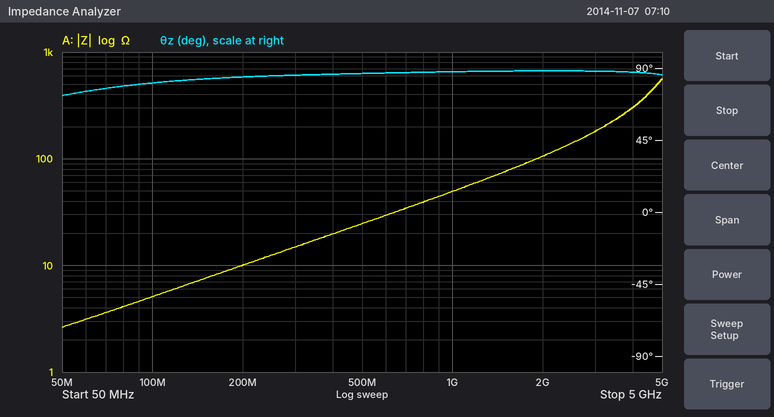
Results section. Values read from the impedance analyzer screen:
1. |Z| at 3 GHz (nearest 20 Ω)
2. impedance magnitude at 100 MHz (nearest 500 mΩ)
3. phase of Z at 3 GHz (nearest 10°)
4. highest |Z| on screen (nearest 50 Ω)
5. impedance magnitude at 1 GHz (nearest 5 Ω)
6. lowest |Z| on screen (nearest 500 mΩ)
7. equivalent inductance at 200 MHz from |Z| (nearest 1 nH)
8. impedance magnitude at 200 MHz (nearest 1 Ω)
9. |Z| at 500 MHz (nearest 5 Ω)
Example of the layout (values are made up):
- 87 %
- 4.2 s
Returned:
- 180 Ω
- 5.0 Ω
- 90°
- 550 Ω
- 50 Ω
- 2.5 Ω
- 8 nH
- 10 Ω
- 25 Ω
